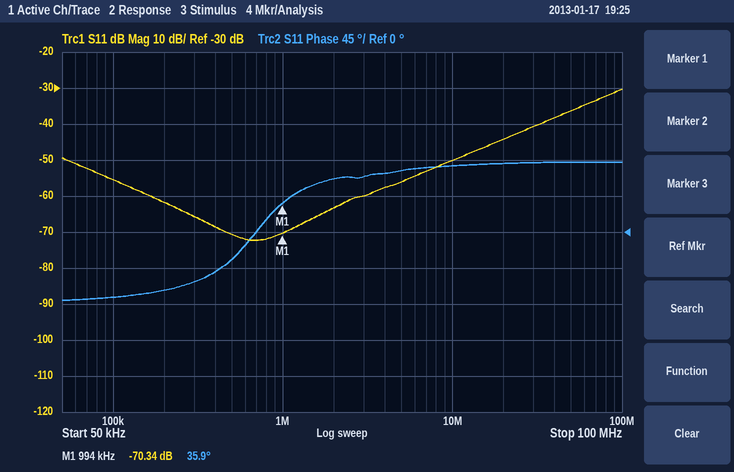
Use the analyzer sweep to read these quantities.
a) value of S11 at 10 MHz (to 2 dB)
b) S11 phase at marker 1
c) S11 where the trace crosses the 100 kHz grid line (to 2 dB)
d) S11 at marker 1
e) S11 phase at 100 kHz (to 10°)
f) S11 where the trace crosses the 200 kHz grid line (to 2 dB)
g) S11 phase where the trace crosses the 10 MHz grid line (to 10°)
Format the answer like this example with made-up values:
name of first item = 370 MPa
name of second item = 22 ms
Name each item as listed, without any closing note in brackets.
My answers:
value of S11 at 10 MHz = -50 dB
S11 phase at marker 1 = 35.9°
S11 where the trace crosses the 100 kHz grid line = -56 dB
S11 at marker 1 = -70.34 dB
S11 phase at 100 kHz = -80°
S11 where the trace crosses the 200 kHz grid line = -62 dB
S11 phase where the trace crosses the 10 MHz grid line = 80°
